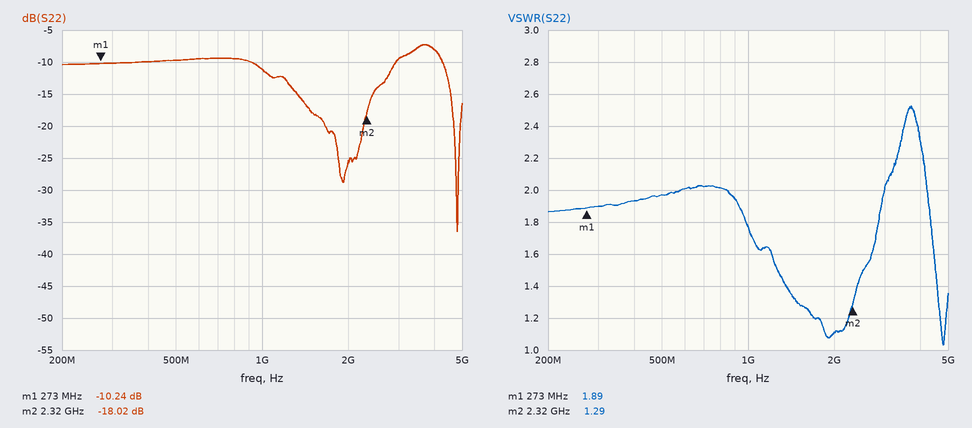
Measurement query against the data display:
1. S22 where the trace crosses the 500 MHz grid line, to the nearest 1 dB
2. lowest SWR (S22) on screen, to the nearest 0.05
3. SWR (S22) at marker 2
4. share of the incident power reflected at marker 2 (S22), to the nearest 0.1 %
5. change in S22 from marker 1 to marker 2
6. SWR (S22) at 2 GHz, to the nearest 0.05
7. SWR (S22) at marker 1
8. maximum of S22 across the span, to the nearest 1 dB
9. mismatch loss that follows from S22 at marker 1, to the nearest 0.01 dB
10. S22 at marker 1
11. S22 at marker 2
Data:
-10 dB
1.05
1.29
1.6 %
-7.78 dB
1.10
1.89
-7 dB
0.43 dB
-10.24 dB
-18.02 dB
